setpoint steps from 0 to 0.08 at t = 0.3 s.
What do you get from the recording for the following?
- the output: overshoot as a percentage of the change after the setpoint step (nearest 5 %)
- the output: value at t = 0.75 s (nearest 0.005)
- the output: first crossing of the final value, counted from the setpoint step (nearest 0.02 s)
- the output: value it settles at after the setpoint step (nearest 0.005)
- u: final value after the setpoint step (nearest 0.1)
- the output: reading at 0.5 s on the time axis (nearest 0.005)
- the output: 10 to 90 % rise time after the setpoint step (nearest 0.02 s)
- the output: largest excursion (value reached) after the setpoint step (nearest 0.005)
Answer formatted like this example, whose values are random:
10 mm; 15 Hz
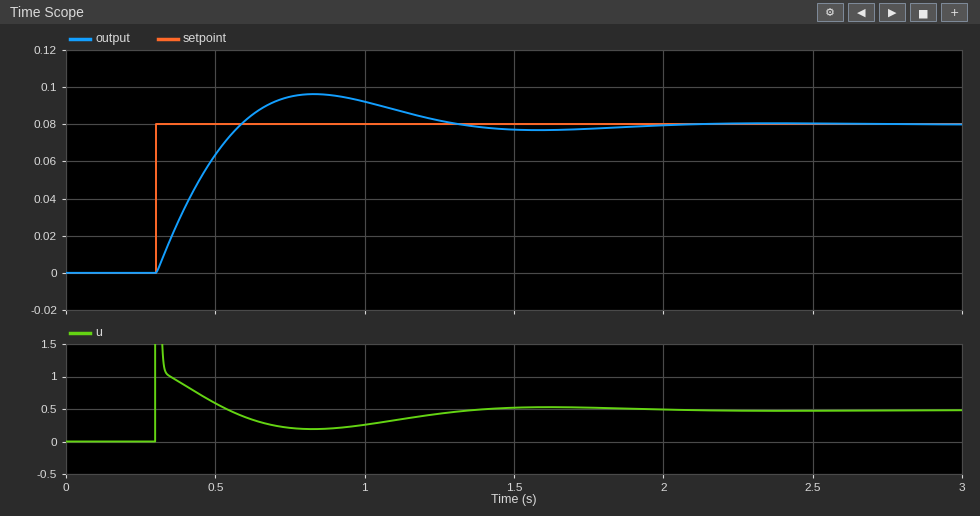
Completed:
20 %; 0.095; 0.28 s; 0.080; 0.5; 0.065; 0.22 s; 0.095
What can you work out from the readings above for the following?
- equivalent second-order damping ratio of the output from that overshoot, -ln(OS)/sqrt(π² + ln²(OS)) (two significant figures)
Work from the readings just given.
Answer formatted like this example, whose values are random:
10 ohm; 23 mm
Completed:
0.46
